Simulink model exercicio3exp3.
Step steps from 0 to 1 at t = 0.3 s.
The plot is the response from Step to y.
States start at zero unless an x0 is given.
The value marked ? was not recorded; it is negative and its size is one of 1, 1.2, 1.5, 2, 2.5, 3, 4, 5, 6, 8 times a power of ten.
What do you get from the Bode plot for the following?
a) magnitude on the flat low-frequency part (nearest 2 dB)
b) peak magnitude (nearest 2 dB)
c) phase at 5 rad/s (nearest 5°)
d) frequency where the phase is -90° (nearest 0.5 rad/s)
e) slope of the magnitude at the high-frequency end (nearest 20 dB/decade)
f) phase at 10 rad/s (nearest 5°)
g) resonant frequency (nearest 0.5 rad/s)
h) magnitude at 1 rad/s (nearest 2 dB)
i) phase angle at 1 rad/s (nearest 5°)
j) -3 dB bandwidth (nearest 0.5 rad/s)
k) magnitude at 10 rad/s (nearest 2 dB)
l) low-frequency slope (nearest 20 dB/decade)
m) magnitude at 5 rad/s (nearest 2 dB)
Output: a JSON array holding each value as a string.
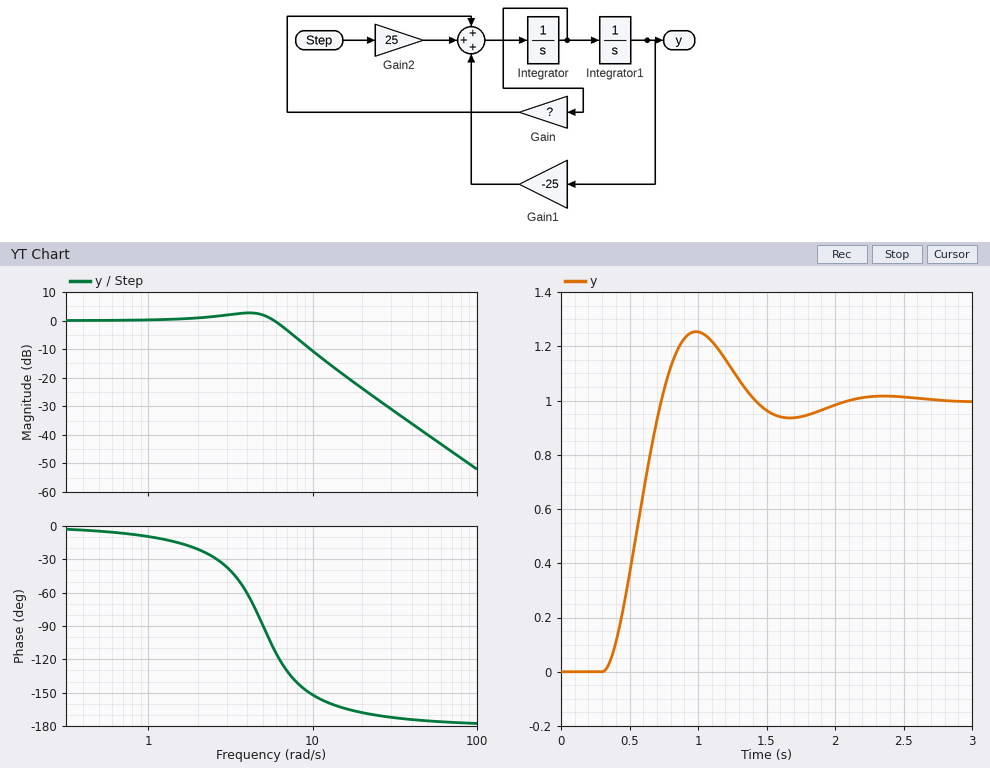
["0 dB", "2 dB", "-90°", "5.0 rad/s", "-40 dB/decade", "-150°", "4.0 rad/s", "0 dB", "-10°", "7.0 rad/s", "-10 dB", "0 dB/decade", "2 dB"]
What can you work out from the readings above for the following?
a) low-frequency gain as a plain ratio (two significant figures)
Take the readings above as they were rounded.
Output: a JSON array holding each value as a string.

["1.0"]
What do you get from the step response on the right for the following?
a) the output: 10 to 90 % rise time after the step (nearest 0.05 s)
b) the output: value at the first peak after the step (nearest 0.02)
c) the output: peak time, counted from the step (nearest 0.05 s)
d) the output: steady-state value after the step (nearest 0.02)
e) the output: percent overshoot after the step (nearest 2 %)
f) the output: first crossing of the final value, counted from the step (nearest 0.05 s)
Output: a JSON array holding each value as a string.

["0.30 s", "1.26", "0.70 s", "1.00", "26 %", "0.45 s"]
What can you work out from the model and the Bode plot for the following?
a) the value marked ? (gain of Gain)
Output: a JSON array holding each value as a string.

["-4"]
